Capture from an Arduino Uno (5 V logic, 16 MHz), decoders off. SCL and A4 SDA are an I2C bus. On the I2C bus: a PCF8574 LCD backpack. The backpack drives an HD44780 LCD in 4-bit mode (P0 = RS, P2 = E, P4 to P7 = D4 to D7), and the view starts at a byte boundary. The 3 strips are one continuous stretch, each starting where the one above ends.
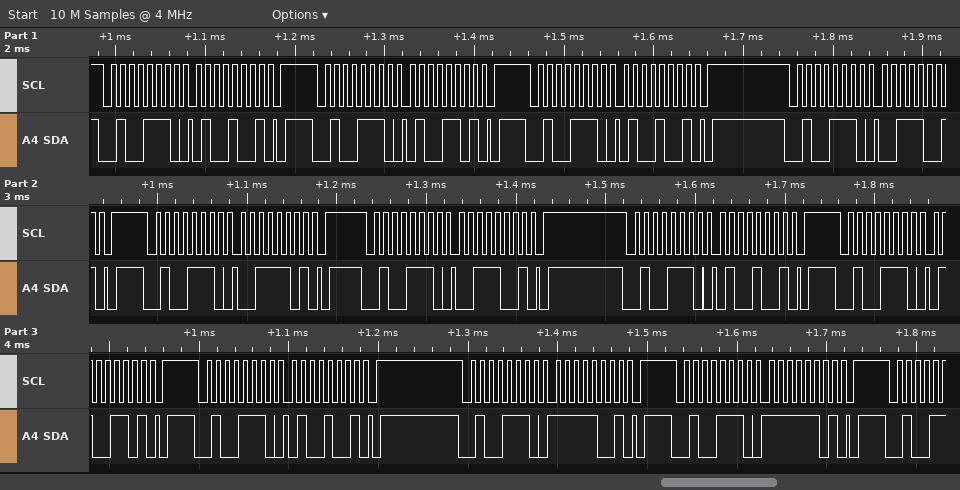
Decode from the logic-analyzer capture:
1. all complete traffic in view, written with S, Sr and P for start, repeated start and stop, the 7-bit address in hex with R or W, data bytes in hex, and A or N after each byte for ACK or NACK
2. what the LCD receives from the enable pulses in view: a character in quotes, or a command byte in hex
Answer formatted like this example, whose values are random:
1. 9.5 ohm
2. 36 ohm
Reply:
1. S 27W A 49 A P S 27W A 4D A P S 27W A 49 A P S 27W A 39 A P S 27W A 3D A P S 27W A 39 A P S 27W A 49 A P S 27W A 4D A P S 27W A 49 A P S 27W A F9 A P S 27W A FD A P
2. 'C'
